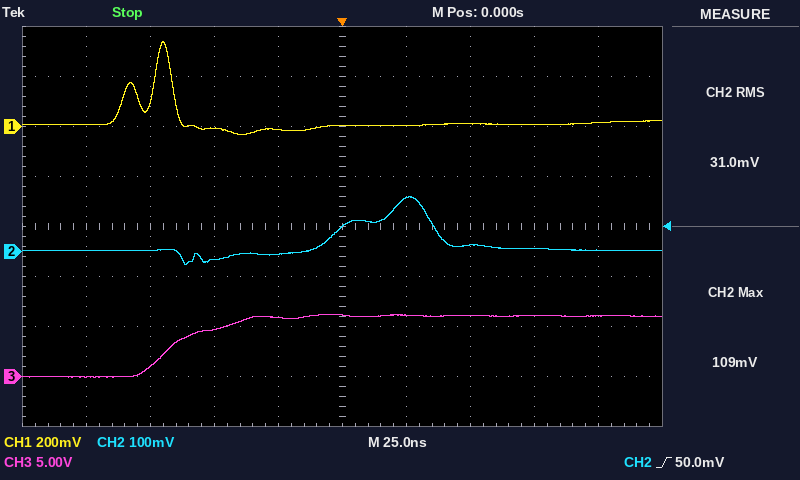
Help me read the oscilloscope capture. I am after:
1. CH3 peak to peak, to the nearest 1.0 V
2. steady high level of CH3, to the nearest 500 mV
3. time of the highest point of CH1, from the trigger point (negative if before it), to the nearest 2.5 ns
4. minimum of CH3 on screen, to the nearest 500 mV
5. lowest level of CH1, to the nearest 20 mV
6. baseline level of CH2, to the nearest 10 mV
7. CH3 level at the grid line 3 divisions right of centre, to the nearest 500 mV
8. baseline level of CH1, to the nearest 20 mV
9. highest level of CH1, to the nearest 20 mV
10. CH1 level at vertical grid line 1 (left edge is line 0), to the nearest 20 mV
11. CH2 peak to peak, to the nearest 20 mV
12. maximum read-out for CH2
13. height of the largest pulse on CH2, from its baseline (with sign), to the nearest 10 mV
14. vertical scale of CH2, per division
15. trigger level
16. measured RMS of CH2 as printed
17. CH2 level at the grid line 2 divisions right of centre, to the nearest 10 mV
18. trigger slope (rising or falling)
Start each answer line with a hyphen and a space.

- 6.0 V
- 6.0 V
- -70.0 ns
- 0.0 V
- -40 mV
- 0 mV
- 6.0 V
- 0 mV
- 340 mV
- 0 mV
- 140 mV
- 109 mV
- +110 mV
- 100 mV
- 50.0 mV
- 31.0 mV
- 10 mV
- rising
